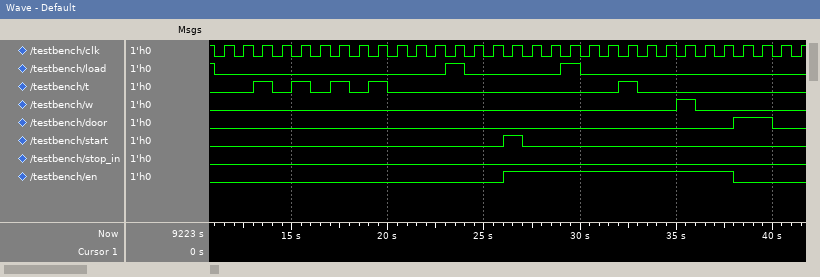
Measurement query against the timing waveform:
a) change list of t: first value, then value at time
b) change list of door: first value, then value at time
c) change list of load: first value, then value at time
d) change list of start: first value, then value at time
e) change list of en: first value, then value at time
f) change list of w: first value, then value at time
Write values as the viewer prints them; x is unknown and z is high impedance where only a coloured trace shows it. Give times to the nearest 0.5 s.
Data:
0, 1 at 13 s, 0 at 14 s, 1 at 15 s, 0 at 16 s, 1 at 17 s, 0 at 18 s, 1 at 19 s, 0 at 20 s, 1 at 32 s, 0 at 33 s
0, 1 at 38 s, 0 at 40 s
1, 0 at 11 s, 1 at 23 s, 0 at 24 s, 1 at 29 s, 0 at 30 s
0, 1 at 26 s, 0 at 27 s
0, 1 at 26 s, 0 at 38 s
0, 1 at 35 s, 0 at 36 s
